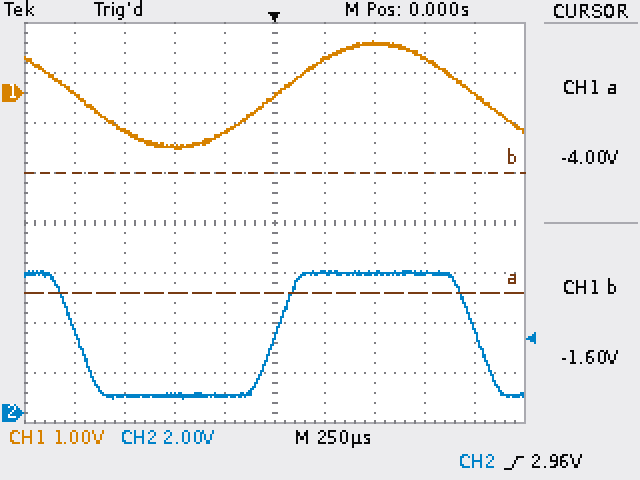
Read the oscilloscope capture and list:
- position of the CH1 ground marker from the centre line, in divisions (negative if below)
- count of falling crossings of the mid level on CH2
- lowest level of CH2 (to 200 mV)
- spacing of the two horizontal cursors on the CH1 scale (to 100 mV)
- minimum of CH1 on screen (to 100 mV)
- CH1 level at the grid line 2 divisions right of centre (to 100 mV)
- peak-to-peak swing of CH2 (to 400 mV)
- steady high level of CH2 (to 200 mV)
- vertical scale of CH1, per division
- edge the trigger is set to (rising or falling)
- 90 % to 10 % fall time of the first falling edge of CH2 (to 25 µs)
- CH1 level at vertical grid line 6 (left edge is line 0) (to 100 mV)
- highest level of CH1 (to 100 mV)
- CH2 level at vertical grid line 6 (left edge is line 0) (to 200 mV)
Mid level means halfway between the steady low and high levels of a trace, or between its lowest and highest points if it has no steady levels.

+2.6 div
2
600 mV
2.4 V
-1.1 V
1.0 V
5.2 V
5.6 V
1 V
rising
200 µs
700 mV
1.0 V
5.6 V
